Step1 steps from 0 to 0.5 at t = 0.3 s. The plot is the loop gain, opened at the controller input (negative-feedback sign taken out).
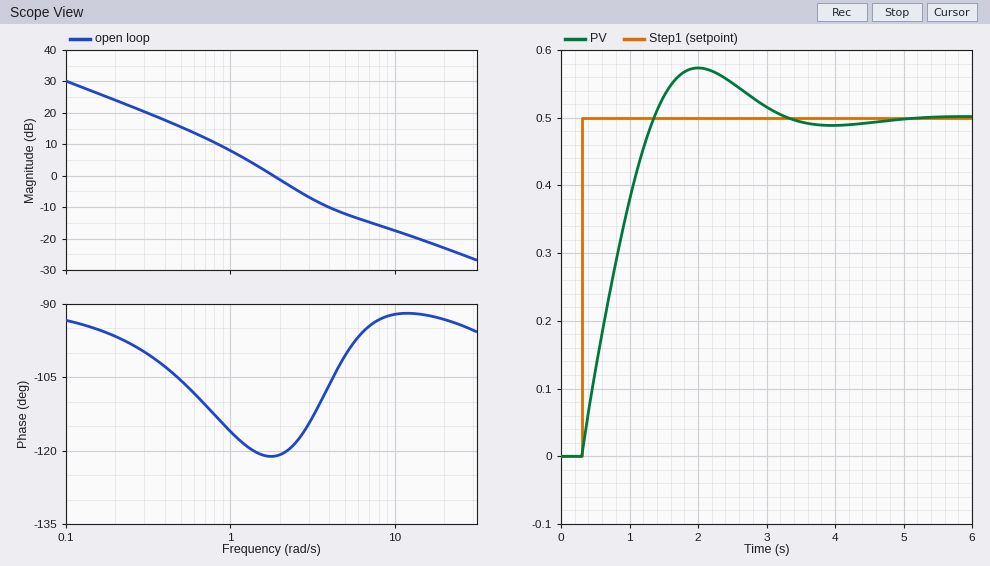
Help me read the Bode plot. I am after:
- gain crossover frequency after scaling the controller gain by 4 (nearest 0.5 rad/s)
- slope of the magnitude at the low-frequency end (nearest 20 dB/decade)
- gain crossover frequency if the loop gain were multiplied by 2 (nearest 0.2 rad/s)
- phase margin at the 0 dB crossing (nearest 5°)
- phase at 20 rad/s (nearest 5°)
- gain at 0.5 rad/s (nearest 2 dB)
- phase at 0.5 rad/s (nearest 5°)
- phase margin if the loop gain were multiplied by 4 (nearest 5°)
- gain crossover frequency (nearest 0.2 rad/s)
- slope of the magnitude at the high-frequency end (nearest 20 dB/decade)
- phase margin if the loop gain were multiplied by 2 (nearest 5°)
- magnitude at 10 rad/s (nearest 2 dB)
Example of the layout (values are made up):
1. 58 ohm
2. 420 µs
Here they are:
1. 5.0 rad/s
2. -20 dB/decade
3. 2.8 rad/s
4. 60°
5. -95°
6. 16 dB
7. -105°
8. 80°
9. 1.8 rad/s
10. -20 dB/decade
11. 65°
12. -18 dB
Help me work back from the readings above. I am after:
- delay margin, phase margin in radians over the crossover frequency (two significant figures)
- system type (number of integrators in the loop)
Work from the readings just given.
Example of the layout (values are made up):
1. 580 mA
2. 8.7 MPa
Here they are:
1. 0.58 s
2. 1
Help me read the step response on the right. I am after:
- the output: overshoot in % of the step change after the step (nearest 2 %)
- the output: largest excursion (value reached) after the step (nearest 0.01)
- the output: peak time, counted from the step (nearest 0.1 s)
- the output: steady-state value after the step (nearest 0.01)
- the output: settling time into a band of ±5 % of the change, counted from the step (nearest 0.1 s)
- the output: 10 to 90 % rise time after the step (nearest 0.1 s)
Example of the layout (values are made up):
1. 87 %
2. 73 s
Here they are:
1. 14 %
2. 0.57
3. 1.7 s
4. 0.50
5. 2.6 s
6. 0.8 s
